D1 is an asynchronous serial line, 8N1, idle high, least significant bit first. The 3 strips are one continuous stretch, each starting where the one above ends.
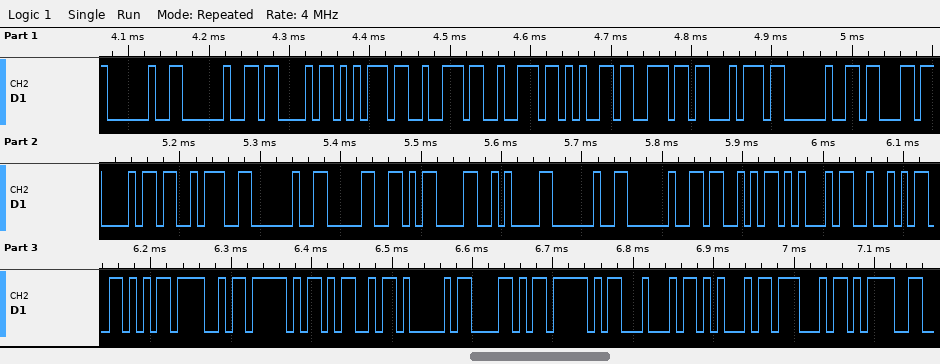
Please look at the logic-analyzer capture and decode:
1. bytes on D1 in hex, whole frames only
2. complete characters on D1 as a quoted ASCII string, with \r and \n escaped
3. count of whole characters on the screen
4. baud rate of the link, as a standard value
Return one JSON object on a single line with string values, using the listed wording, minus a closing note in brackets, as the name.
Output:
{"bytes on D1 in hex, whole frames only": "0x20 0x20 0x43 0x75 0x72 0x72 0x65 0x6E 0x74 0x20 0x63 0x68 0x3A 0x20 0x30 0x0D 0x0A 0x20 0x20 0x53 0x45 0x52 0x56 0x4F 0x5F 0x4D 0x41 0x58 0x5F 0x44 0x45 0x47 0x3D", "complete characters on D1 as a quoted ASCII string, with \\r and \\n escaped": "\"  Current ch: 0\\r\\n  SERVO_MAX_DEG=\"", "count of whole characters on the screen": "33", "baud rate of the link, as a standard value": "115200 baud"}
